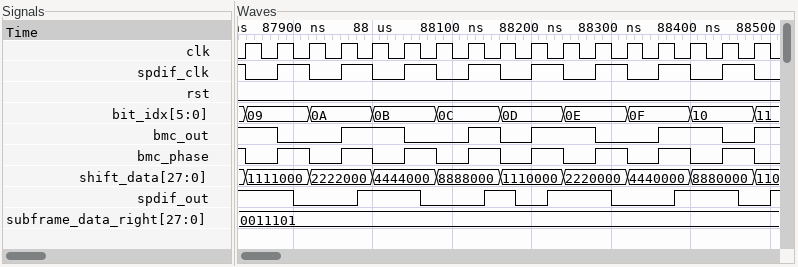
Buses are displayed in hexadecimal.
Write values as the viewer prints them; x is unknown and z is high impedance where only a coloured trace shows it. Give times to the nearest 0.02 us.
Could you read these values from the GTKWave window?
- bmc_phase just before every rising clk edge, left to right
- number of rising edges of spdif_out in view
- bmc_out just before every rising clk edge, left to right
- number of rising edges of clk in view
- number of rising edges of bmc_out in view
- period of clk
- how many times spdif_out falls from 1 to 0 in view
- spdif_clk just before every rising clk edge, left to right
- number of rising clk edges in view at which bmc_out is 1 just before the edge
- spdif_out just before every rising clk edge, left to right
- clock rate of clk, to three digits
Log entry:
1 0 1 0 1 0 1 0 1 0 1 0 1 0 1 0 1
5
1 1 0 0 1 1 0 0 1 0 1 1 0 0 1 1 0
17
5
0.04 us
5
1 0 1 0 1 0 1 0 1 0 1 0 1 0 1 0 1
9
1 1 0 0 1 1 0 0 1 0 1 1 0 0 1 1 0
25.0 MHz
